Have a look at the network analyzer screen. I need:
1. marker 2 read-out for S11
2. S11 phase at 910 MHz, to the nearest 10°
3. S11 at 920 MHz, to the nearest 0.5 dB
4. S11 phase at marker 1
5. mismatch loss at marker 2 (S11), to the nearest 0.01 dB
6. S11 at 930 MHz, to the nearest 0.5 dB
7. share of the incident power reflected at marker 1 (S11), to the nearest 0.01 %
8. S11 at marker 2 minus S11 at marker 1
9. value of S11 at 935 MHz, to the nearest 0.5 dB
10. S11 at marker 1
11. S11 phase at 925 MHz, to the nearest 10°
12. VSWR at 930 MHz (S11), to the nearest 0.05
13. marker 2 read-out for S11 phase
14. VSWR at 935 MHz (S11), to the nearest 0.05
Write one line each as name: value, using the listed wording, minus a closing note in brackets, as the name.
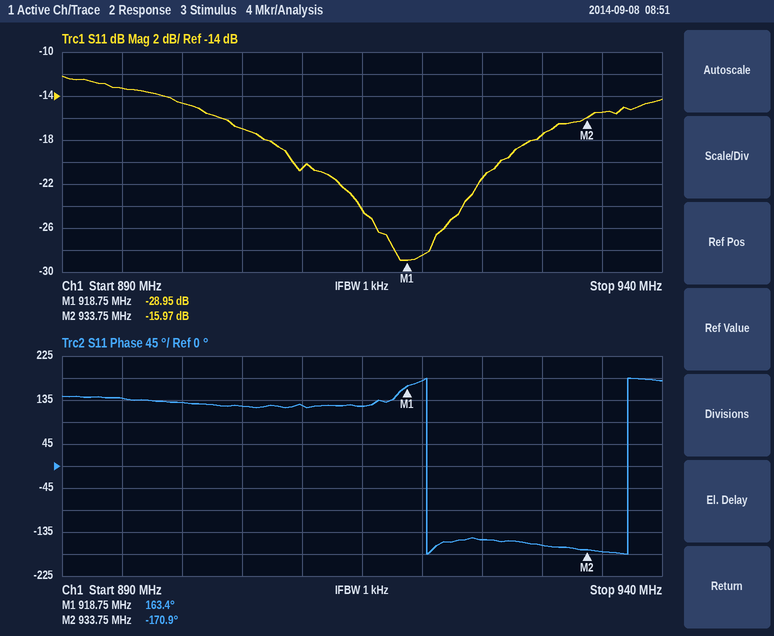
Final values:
marker 2 read-out for S11: -15.97 dB
S11 phase at 910 MHz, to the nearest 10°: 120°
S11 at 920 MHz, to the nearest 0.5 dB: -28.5 dB
S11 phase at marker 1: 163.4°
mismatch loss at marker 2 (S11), to the nearest 0.01 dB: 0.11 dB
S11 at 930 MHz, to the nearest 0.5 dB: -17.5 dB
share of the incident power reflected at marker 1 (S11), to the nearest 0.01 %: 0.13 %
S11 at marker 2 minus S11 at marker 1: 12.98 dB
value of S11 at 935 MHz, to the nearest 0.5 dB: -15.5 dB
S11 at marker 1: -28.95 dB
S11 phase at 925 MHz, to the nearest 10°: -150°
VSWR at 930 MHz (S11), to the nearest 0.05: 1.30
marker 2 read-out for S11 phase: -170.9°
VSWR at 935 MHz (S11), to the nearest 0.05: 1.40
